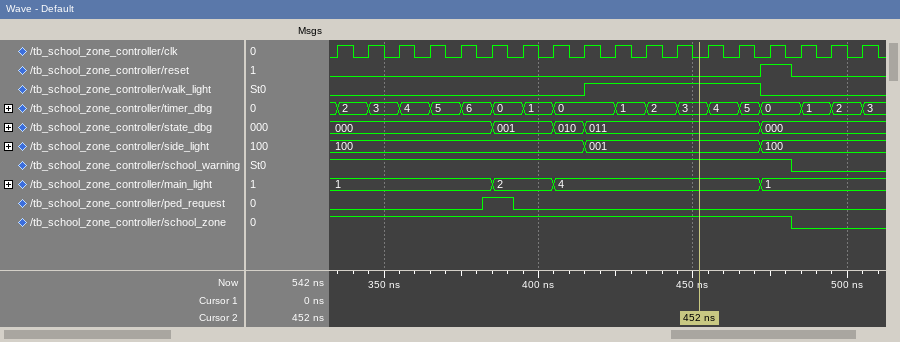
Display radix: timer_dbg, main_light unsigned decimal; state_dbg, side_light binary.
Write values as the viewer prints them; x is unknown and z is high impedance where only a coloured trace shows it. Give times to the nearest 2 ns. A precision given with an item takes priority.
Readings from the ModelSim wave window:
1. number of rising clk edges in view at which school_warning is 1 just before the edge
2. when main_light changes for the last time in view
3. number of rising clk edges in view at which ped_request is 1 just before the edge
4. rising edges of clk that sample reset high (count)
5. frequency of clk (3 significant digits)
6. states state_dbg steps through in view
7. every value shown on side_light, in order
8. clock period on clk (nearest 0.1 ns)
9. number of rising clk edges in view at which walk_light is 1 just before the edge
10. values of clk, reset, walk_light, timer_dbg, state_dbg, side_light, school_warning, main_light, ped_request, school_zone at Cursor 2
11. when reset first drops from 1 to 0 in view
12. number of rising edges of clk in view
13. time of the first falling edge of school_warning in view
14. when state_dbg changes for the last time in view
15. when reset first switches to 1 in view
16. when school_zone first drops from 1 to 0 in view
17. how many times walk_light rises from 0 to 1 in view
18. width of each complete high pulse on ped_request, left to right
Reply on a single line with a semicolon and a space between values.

15; 472 ns; 1; 1; 100 MHz; 000, 001, 010, 011, 000; 100, 001, 100; 10 ns; 5; clk=0, reset=0, walk_light=1, timer_dbg=3, state_dbg=011, side_light=001, school_warning=1, main_light=4, ped_request=0, school_zone=1; 482 ns; 18; 482 ns; 472 ns; 472 ns; 482 ns; 1; 10 ns
